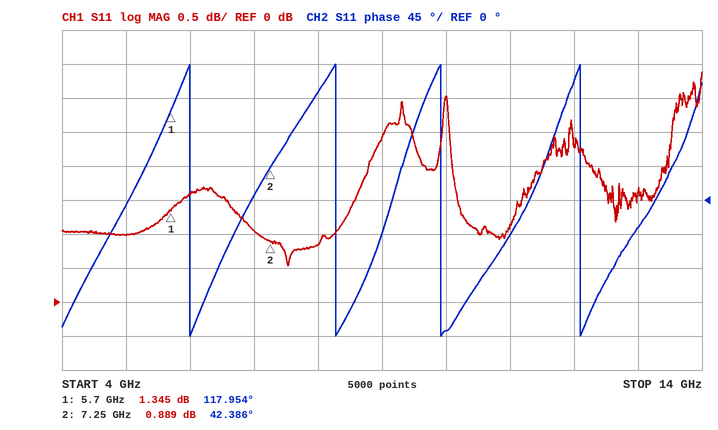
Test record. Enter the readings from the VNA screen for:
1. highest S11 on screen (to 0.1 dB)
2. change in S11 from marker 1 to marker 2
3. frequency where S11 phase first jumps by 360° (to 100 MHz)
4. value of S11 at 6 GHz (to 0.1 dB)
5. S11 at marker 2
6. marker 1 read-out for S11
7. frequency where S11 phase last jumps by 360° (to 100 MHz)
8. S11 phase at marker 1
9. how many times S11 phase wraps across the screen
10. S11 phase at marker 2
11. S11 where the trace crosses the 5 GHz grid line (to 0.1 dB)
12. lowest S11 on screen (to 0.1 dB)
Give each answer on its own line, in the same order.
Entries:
3.4 dB
-0.456 dB
6.0 GHz
1.6 dB
0.889 dB
1.345 dB
12.1 GHz
117.954°
4
42.386°
1.0 dB
0.5 dB
